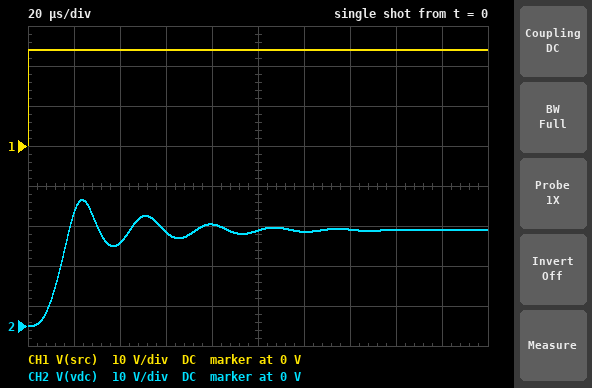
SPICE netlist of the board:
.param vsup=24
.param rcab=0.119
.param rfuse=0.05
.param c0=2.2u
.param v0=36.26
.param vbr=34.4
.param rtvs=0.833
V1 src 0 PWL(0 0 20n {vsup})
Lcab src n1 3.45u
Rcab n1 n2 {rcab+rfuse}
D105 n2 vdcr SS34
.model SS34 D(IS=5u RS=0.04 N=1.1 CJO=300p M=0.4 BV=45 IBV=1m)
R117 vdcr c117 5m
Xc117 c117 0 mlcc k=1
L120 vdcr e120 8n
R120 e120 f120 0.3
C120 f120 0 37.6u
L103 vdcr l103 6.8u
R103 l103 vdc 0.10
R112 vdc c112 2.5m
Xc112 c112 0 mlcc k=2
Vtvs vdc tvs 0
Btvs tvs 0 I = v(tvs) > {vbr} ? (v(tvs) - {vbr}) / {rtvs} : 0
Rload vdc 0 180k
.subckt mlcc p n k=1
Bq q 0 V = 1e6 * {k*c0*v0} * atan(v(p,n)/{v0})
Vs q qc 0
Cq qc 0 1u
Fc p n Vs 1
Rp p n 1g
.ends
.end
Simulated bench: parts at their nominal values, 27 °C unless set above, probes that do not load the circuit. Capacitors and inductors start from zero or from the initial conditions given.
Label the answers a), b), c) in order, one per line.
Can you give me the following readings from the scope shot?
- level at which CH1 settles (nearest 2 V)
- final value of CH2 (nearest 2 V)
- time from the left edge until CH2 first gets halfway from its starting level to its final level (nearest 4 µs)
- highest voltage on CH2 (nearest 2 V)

a) 24 V
b) 24 V
c) 12 µs
d) 32 V
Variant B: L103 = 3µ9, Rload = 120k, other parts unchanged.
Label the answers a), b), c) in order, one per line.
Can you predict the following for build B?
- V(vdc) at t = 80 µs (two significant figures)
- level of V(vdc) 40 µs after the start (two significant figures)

a) 24 V
b) 26 V
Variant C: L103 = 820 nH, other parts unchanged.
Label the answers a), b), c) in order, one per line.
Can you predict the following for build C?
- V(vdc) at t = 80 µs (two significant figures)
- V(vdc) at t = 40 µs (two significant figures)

a) 24 V
b) 25 V
